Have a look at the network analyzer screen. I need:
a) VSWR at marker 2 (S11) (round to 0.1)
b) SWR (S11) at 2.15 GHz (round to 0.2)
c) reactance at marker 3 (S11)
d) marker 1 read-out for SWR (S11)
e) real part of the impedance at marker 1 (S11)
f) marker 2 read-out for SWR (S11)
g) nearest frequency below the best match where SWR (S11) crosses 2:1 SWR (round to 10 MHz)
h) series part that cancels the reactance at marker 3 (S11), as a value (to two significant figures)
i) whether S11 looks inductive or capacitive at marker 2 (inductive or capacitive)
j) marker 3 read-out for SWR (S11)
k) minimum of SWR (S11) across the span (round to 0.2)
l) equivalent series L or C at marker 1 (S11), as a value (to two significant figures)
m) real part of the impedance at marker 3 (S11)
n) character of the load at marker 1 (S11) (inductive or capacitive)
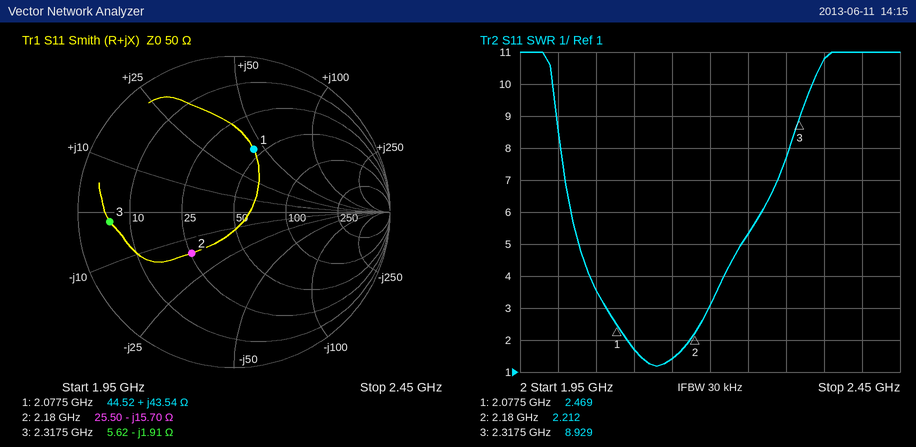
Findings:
2.2
1.4
-1.91 Ω
2.469
44.52 Ω
2.212
2.09 GHz
130 pH
capacitive
8.929
1.2
3.3 nH
5.62 Ω
inductive
